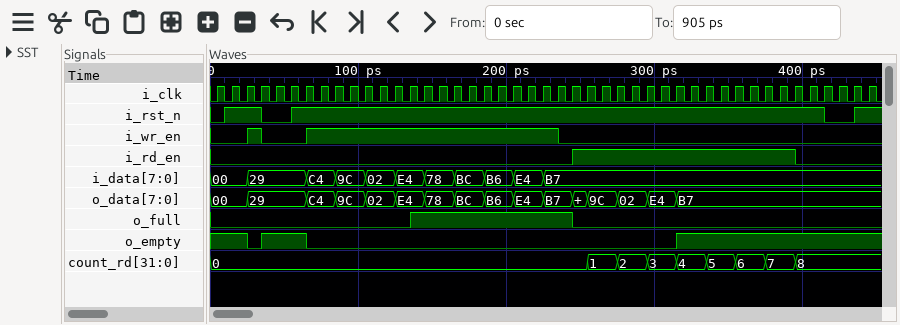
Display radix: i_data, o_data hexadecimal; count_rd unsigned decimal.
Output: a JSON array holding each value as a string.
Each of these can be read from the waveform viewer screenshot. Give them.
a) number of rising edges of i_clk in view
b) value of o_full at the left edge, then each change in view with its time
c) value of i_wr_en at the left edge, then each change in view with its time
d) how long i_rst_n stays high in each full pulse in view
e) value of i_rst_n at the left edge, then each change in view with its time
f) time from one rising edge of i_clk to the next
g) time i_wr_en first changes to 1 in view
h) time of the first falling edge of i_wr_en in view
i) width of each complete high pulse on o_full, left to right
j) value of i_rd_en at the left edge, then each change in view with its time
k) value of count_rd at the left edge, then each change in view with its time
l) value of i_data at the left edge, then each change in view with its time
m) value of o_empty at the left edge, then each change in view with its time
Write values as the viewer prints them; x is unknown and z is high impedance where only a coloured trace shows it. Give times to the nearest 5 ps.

["45", "0, 1 at 135 ps, 0 at 245 ps", "0, 1 at 25 ps, 0 at 35 ps, 1 at 65 ps, 0 at 235 ps", "25 ps, 360 ps", "0, 1 at 10 ps, 0 at 35 ps, 1 at 55 ps, 0 at 415 ps, 1 at 435 ps", "10 ps", "25 ps", "35 ps", "110 ps", "0, 1 at 245 ps, 0 at 395 ps", "0, 1 at 255 ps, 2 at 275 ps, 3 at 295 ps, 4 at 315 ps, 5 at 335 ps, 6 at 355 ps, 7 at 375 ps, 8 at 395 ps", "00, 29 at 25 ps, C4 at 65 ps, 9C at 85 ps, 02 at 105 ps, E4 at 125 ps, 78 at 145 ps, BC at 165 ps, B6 at 185 ps, E4 at 205 ps, B7 at 225 ps", "1, 0 at 25 ps, 1 at 35 ps, 0 at 65 ps, 1 at 315 ps"]
